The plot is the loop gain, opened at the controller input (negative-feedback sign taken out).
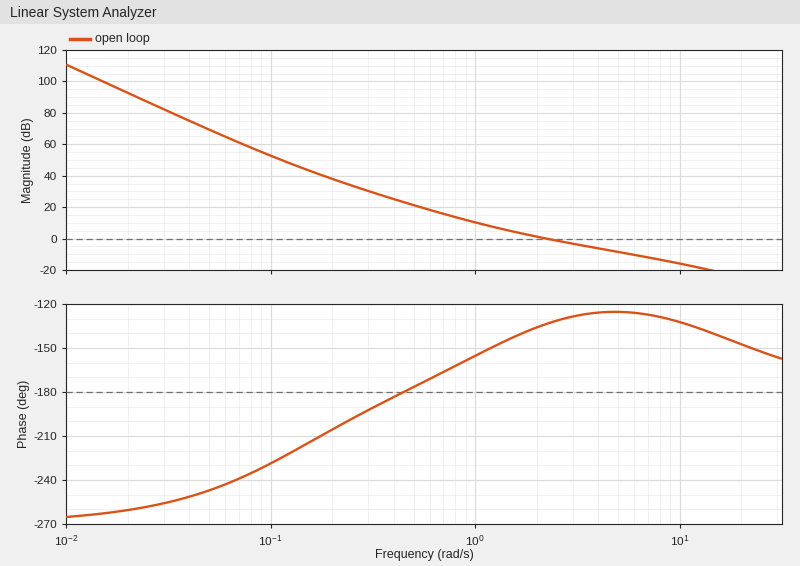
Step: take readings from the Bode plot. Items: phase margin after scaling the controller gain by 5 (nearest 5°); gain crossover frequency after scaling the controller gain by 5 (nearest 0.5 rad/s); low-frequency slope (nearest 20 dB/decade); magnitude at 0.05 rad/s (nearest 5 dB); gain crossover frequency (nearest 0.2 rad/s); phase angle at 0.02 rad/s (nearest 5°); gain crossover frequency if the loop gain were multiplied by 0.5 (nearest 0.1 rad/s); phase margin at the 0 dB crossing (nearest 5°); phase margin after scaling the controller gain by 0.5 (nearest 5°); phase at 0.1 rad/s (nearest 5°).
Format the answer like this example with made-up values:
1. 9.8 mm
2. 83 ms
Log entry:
1. 50°
2. 8.5 rad/s
3. -60 dB/decade
4. 70 dB
5. 2.2 rad/s
6. -260°
7. 1.4 rad/s
8. 45°
9. 35°
10. -230°
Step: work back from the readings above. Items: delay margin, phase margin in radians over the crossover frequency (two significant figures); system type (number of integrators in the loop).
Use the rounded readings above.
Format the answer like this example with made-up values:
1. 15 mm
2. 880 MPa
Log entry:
1. 0.36 s
2. 3
